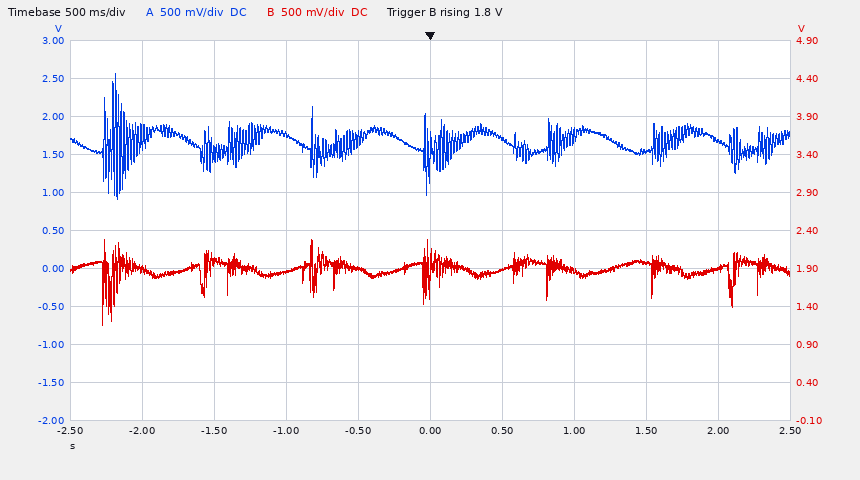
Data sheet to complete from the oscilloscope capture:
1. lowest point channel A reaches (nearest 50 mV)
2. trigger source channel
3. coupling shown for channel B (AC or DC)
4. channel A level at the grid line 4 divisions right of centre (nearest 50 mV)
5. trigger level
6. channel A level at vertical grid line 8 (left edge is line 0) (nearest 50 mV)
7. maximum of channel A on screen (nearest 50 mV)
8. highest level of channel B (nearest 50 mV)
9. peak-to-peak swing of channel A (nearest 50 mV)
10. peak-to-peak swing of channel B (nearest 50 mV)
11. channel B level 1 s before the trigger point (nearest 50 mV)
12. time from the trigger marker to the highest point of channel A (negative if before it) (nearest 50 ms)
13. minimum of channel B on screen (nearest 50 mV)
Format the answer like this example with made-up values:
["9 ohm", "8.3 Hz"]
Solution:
["900 mV", "channel B", "DC", "1.70 V", "1.8 V", "1.55 V", "2.55 V", "2.30 V", "1.65 V", "1.15 V", "1.85 V", "-2.20 s", "1.15 V"]
